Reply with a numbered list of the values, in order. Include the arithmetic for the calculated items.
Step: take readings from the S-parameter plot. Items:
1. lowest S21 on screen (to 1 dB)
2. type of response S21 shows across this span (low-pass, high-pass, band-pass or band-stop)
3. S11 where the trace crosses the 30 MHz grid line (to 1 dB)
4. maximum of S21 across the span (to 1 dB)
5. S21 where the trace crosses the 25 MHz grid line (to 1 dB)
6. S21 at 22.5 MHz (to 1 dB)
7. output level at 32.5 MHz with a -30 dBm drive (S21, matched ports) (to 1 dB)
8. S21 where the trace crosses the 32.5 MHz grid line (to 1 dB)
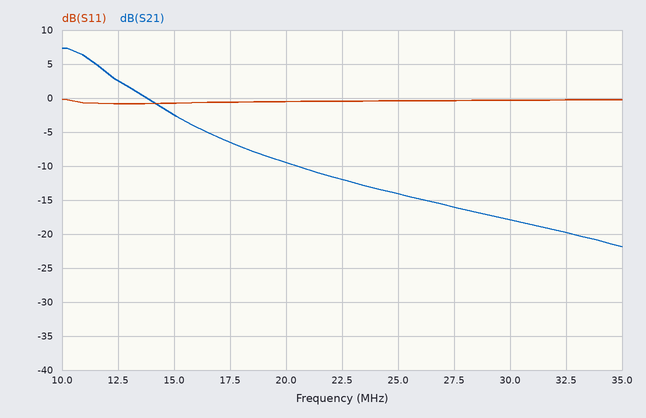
1. -22 dB
2. low-pass
3. 0 dB
4. 7 dB
5. -14 dB
6. -12 dB
7. -30 dBm + (-20 dB) = -50 dBm
8. -20 dB
